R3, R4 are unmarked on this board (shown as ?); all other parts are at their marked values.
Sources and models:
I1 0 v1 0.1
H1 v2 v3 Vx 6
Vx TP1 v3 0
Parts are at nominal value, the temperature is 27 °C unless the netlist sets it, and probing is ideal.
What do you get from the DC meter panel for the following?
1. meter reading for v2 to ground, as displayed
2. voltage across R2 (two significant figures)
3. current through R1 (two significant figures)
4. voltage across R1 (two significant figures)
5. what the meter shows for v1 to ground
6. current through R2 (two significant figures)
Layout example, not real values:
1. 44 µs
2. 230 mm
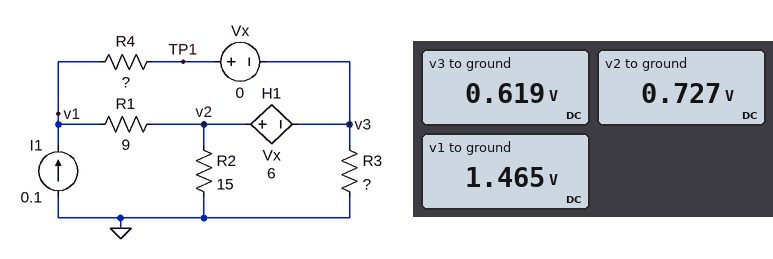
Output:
1. 0.727 V
2. 730 mV
3. 82 mA
4. 740 mV
5. 1.465 V
6. 48 mA
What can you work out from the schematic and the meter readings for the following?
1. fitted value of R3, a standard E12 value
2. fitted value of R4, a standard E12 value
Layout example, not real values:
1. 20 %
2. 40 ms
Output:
1. 12 Ω
2. 47 Ω
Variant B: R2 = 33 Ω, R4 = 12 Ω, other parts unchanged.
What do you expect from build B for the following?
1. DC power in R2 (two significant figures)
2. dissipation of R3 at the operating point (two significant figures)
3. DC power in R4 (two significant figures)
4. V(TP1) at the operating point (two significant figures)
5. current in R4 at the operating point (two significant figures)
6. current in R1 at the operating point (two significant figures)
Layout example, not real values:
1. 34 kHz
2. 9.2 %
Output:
1. 40 mW
2. 51 mW
3. 43 mW
4. 780 mV
5. 60 mA
6. 40 mA
